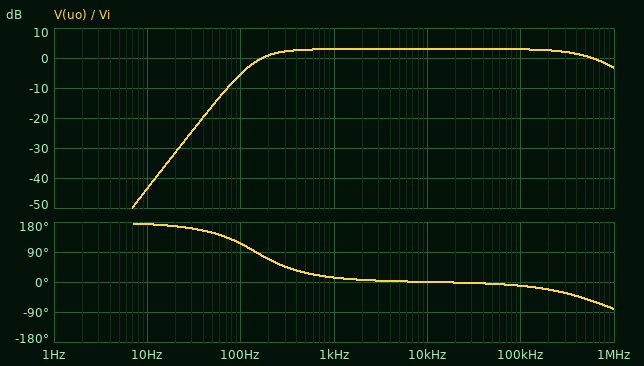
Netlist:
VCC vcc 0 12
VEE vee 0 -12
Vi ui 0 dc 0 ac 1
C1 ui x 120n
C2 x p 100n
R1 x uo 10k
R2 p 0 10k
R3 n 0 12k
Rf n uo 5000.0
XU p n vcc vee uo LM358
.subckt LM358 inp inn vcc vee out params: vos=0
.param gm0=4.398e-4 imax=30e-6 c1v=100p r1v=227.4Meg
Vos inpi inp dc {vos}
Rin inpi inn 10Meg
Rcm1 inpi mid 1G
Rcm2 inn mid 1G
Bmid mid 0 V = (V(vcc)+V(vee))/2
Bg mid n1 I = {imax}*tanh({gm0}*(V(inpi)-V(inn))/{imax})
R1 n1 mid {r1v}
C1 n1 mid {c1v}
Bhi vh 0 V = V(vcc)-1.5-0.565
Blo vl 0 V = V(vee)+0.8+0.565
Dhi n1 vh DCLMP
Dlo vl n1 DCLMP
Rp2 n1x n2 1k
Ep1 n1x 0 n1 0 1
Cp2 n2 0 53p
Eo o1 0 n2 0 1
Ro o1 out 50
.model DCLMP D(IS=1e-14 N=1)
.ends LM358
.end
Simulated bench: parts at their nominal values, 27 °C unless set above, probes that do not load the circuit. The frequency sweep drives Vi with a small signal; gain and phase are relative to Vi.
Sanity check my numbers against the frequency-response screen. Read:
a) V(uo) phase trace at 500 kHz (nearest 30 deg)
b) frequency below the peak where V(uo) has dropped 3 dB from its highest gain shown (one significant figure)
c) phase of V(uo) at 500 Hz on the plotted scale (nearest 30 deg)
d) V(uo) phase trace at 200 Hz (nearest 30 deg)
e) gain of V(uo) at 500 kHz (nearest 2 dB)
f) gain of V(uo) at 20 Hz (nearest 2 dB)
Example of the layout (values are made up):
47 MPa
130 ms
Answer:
-60 deg
200 Hz
30 deg
60 deg
0 dB
-32 dB
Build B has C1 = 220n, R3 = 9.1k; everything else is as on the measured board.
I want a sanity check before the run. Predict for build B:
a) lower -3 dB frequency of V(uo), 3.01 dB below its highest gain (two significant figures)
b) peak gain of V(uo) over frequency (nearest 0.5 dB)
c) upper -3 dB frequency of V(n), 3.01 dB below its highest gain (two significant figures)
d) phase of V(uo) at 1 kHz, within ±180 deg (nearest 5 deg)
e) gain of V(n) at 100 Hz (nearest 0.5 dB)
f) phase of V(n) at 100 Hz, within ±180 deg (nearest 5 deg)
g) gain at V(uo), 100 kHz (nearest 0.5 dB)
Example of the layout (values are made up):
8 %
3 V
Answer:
140 Hz
4.0 dB
520 kHz
10 deg
-5.5 dB
95 deg
3.5 dB
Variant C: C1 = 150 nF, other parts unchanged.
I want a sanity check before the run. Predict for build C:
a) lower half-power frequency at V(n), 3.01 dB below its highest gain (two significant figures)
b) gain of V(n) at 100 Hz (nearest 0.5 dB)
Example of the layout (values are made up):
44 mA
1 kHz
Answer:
160 Hz
-7.5 dB
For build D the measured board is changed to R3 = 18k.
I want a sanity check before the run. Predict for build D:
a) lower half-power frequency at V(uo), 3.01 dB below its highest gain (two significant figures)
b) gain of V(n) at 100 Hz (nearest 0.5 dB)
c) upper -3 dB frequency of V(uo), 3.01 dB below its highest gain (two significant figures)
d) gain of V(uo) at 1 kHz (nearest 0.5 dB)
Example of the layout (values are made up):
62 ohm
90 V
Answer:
190 Hz
-9.0 dB
660 kHz
2.0 dB
